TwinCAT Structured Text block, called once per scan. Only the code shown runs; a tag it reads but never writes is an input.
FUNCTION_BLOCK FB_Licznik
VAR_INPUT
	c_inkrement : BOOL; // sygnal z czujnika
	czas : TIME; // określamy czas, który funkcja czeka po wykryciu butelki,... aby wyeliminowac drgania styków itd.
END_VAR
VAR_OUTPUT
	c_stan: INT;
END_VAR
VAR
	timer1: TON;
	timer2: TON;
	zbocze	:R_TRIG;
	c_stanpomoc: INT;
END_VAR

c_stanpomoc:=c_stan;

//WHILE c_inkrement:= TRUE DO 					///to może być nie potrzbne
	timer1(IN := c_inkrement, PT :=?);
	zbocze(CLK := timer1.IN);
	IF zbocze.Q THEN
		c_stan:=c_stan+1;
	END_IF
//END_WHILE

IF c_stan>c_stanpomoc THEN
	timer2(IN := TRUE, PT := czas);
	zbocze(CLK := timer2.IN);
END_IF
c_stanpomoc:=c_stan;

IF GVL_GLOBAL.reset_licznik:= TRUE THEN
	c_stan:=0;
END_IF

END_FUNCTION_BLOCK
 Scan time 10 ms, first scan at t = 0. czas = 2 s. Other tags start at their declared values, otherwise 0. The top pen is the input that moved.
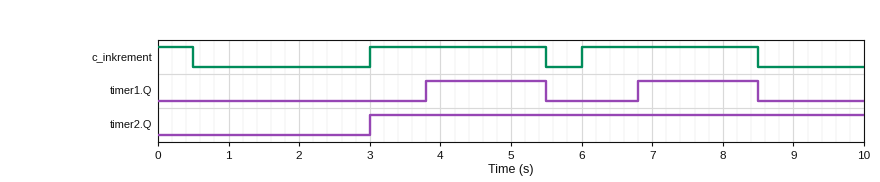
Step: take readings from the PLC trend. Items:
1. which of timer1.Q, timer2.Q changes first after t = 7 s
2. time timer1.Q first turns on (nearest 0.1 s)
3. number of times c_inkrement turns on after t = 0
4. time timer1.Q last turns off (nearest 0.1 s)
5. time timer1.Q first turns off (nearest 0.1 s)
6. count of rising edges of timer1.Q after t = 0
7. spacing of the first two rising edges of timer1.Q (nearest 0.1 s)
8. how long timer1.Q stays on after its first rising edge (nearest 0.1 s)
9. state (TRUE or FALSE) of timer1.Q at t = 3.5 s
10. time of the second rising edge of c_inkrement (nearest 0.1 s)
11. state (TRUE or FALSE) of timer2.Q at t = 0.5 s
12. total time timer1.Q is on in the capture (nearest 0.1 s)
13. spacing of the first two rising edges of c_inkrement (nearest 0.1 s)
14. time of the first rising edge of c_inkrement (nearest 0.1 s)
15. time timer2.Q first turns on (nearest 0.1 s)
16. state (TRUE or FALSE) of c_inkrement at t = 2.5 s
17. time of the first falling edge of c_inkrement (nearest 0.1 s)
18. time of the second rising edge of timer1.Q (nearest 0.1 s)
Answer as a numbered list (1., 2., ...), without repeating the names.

1. timer1.Q
2. 3.8 s
3. 2
4. 8.5 s
5. 5.5 s
6. 2
7. 3.0 s
8. 1.7 s
9. FALSE
10. 6.0 s
11. FALSE
12. 3.4 s
13. 3.0 s
14. 3.0 s
15. 3.0 s
16. FALSE
17. 0.5 s
18. 6.8 s
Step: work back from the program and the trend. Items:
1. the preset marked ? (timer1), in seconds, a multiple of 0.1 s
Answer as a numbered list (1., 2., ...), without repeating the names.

1. 0.8 s
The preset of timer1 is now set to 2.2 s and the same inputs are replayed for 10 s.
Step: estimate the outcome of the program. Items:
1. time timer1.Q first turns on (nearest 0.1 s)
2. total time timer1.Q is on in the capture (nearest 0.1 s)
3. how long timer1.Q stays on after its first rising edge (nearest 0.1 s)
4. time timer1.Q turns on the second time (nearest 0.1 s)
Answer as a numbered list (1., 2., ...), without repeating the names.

1. 5.2 s
2. 0.6 s
3. 0.3 s
4. 8.2 s
